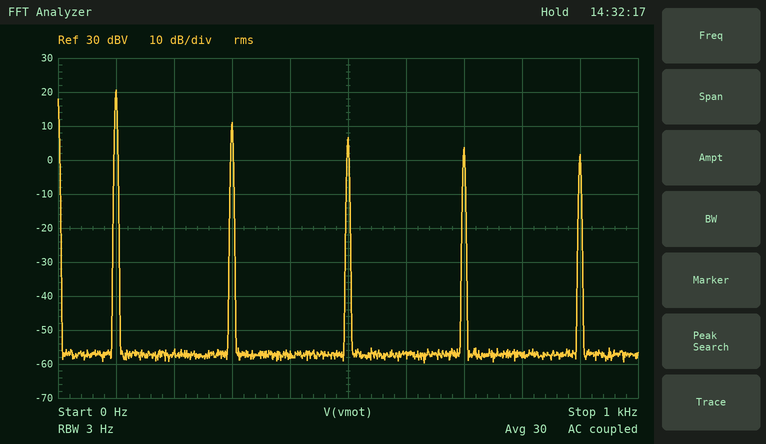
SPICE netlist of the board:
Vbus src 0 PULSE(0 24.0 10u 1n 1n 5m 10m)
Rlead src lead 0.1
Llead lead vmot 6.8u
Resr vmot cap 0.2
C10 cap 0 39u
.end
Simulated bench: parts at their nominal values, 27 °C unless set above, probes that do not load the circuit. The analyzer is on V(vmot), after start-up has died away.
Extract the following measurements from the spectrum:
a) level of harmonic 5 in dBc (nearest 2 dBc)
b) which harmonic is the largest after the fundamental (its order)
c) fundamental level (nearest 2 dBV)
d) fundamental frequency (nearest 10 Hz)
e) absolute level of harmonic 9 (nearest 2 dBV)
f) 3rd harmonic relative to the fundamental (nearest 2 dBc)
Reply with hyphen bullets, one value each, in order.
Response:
- -14 dBc
- 3
- 20 dBV
- 100 Hz
- 2 dBV
- -10 dBc
